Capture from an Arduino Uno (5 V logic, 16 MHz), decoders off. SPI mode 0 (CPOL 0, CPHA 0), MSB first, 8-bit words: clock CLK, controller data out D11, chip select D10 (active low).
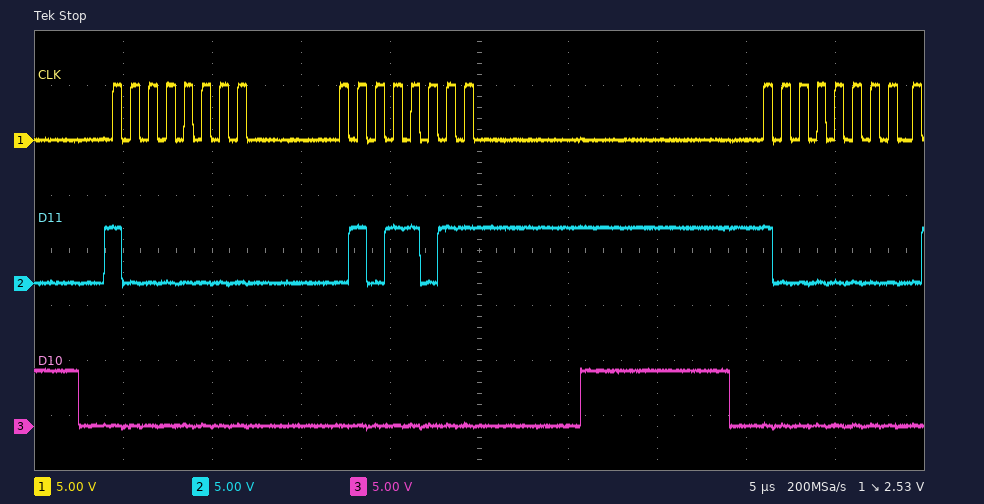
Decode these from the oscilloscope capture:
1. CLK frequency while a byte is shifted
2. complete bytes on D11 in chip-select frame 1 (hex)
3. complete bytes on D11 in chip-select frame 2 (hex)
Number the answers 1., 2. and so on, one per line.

1. 1 MHz
2. 80 5B
3. 80
